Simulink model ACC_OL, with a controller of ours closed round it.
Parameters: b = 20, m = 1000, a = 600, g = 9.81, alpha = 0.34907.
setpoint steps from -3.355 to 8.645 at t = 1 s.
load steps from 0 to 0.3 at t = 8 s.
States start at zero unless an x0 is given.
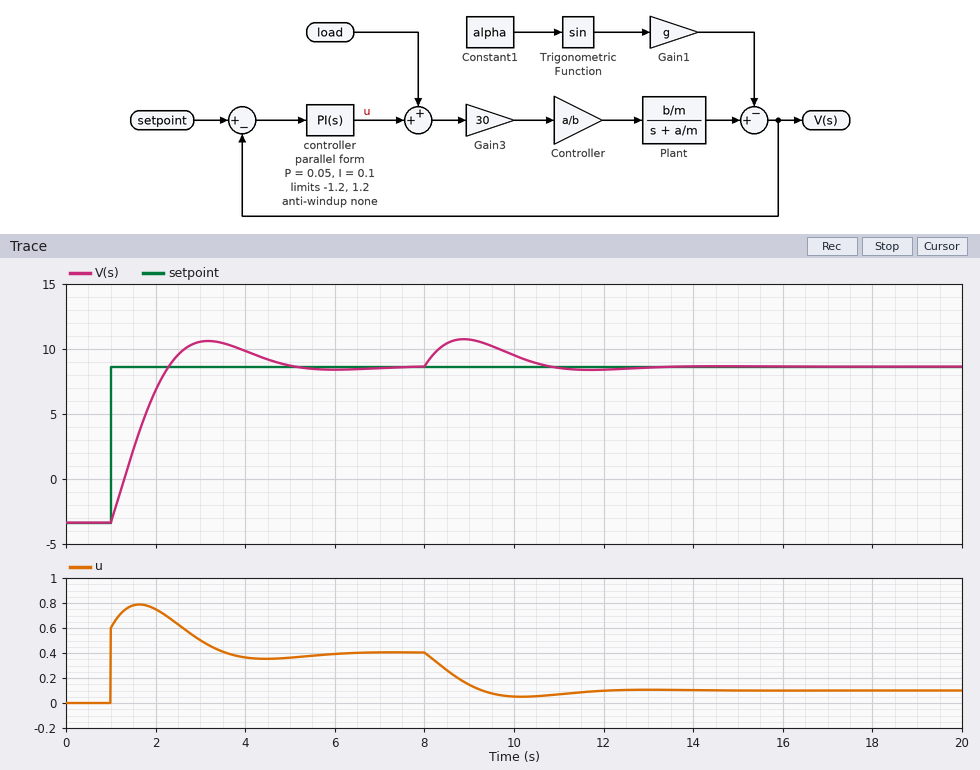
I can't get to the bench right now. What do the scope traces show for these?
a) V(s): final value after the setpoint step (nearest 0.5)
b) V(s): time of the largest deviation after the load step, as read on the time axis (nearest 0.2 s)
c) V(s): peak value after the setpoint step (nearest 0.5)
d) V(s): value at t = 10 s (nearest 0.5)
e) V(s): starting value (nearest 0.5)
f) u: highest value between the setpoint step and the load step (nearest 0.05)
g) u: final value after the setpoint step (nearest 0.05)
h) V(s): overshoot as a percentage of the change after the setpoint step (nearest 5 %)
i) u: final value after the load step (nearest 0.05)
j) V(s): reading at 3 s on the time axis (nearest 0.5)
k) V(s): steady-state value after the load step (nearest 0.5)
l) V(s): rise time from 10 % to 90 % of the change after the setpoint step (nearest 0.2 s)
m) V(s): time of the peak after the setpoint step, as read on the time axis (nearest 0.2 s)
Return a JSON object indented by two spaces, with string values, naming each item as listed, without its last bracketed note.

{
  "V(s): final value after the setpoint step": "8.5",
  "V(s): time of the largest deviation after the load step, as read on the time axis": "8.8 s",
  "V(s): peak value after the setpoint step": "10.5",
  "V(s): value at t = 10 s": "9.5",
  "V(s): starting value": "-3.5",
  "u: highest value between the setpoint step and the load step": "0.80",
  "u: final value after the setpoint step": "0.40",
  "V(s): overshoot as a percentage of the change after the setpoint step": "15 %",
  "u: final value after the load step": "0.10",
  "V(s): reading at 3 s on the time axis": "10.5",
  "V(s): steady-state value after the load step": "8.5",
  "V(s): rise time from 10 % to 90 % of the change after the setpoint step": "1.0 s",
  "V(s): time of the peak after the setpoint step, as read on the time axis": "3.2 s"
}
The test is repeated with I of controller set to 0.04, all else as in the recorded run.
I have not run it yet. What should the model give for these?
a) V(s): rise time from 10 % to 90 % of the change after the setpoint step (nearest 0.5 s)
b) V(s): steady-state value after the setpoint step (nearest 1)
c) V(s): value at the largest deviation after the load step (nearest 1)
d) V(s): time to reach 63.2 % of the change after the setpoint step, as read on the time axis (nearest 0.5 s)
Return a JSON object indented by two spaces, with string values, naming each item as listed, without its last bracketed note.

{
  "V(s): rise time from 10 % to 90 % of the change after the setpoint step": "2.0 s",
  "V(s): steady-state value after the setpoint step": "9",
  "V(s): value at the largest deviation after the load step": "11",
  "V(s): time to reach 63.2 % of the change after the setpoint step, as read on the time axis": "2.0 s"
}
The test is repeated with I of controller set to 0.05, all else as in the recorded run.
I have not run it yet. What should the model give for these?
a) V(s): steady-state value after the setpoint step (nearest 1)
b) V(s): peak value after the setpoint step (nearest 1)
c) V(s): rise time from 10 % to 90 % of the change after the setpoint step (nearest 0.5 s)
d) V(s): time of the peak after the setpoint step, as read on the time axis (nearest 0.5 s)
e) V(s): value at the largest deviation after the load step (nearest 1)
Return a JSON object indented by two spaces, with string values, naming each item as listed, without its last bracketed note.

{
  "V(s): steady-state value after the setpoint step": "9",
  "V(s): peak value after the setpoint step": "9",
  "V(s): rise time from 10 % to 90 % of the change after the setpoint step": "1.5 s",
  "V(s): time of the peak after the setpoint step, as read on the time axis": "4.5 s",
  "V(s): value at the largest deviation after the load step": "11"
}
